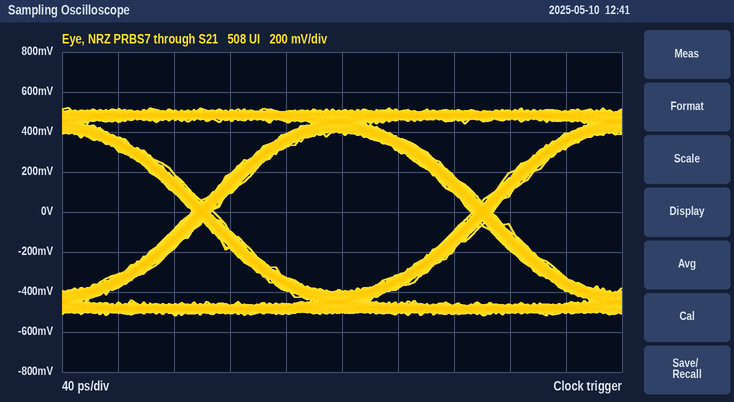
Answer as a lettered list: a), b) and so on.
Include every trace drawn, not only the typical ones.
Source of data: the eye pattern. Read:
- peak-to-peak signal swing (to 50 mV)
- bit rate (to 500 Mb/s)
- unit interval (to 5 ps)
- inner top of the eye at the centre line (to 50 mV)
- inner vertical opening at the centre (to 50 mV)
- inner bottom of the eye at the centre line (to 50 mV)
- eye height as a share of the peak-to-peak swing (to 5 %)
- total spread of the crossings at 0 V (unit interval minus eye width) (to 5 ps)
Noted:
a) 1.05 V
b) 5.0 Gb/s
c) 200 ps
d) 400 mV
e) 800 mV
f) -400 mV
g) 75 %
h) 15 ps
